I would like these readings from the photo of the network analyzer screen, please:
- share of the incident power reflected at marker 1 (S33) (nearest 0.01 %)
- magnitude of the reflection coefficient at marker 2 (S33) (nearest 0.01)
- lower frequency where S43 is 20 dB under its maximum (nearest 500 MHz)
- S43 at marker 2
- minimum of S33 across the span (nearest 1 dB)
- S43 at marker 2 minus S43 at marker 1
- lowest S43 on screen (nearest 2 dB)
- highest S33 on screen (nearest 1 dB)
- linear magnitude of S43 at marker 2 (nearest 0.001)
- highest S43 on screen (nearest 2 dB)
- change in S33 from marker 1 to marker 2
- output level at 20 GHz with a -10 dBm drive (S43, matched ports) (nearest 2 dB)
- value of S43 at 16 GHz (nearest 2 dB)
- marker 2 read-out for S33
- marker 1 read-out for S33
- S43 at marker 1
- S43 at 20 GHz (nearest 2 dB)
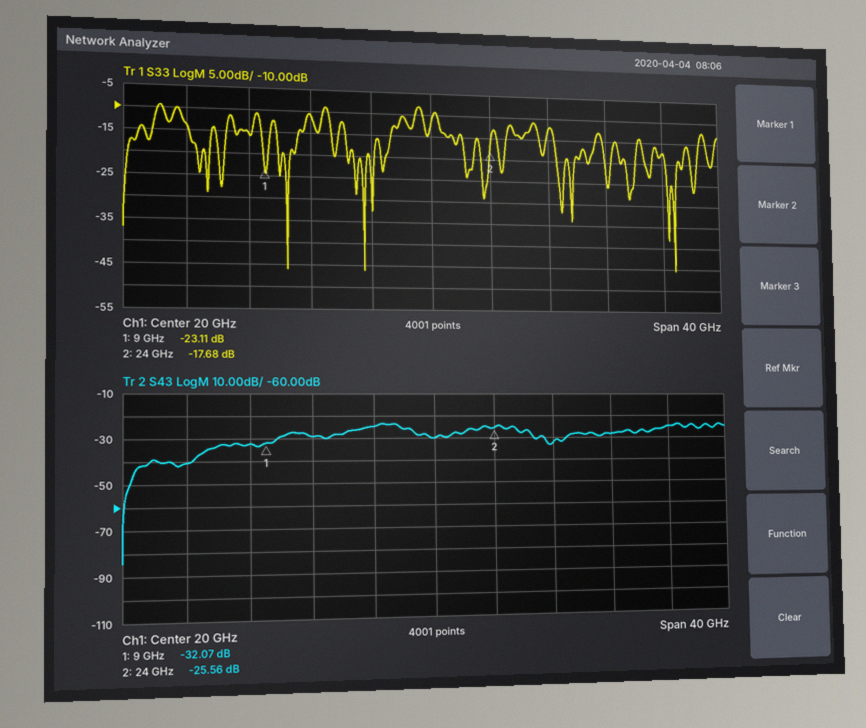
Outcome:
0.49 %
0.13
1.0 GHz
-25.56 dB
-46 dB
6.51 dB
-84 dB
-8 dB
0.053
-24 dB
5.43 dB
-40 dBm
-24 dB
-17.68 dB
-23.11 dB
-32.07 dB
-30 dB
